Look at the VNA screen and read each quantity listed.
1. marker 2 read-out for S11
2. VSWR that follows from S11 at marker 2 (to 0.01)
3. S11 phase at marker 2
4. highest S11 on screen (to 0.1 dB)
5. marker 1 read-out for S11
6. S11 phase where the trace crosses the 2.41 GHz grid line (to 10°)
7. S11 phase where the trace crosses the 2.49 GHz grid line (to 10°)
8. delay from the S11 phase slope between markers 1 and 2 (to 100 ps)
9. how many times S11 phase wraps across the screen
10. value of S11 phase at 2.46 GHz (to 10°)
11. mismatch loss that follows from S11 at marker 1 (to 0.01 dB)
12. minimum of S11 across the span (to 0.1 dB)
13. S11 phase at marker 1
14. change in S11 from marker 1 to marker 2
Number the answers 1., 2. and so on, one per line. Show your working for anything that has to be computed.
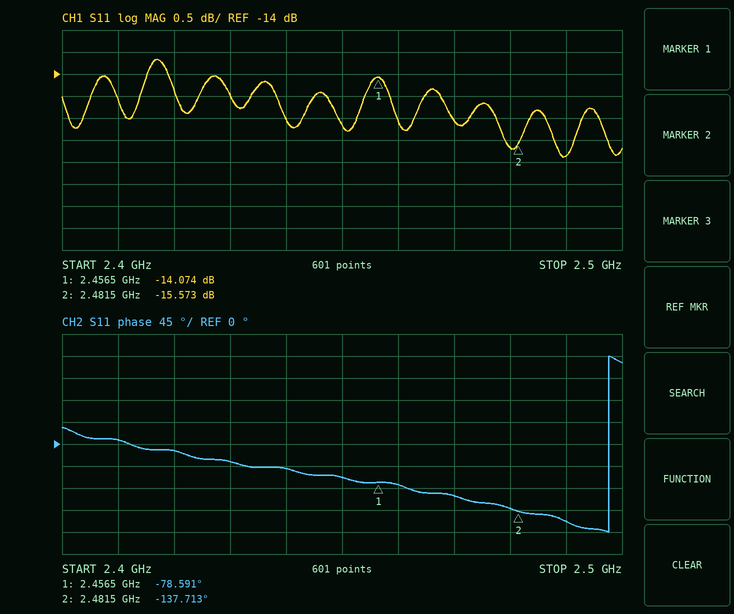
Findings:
1. -15.573 dB
2. (1 + 0.1665)/(1 − 0.1665) ≈ 1.40
3. -137.713°
4. -13.7 dB
5. -14.074 dB
6. 10°
7. -160°
8. −(-137.713° − (-78.591°))/(360° × 25 MHz) ≈ 6.6 ns
9. 1
10. -80°
11. −10 log10(1 − 10^(-14.074/10)) ≈ 0.17 dB
12. -15.9 dB
13. -78.591°
14. -15.573 − (-14.074) = -1.499 dB
